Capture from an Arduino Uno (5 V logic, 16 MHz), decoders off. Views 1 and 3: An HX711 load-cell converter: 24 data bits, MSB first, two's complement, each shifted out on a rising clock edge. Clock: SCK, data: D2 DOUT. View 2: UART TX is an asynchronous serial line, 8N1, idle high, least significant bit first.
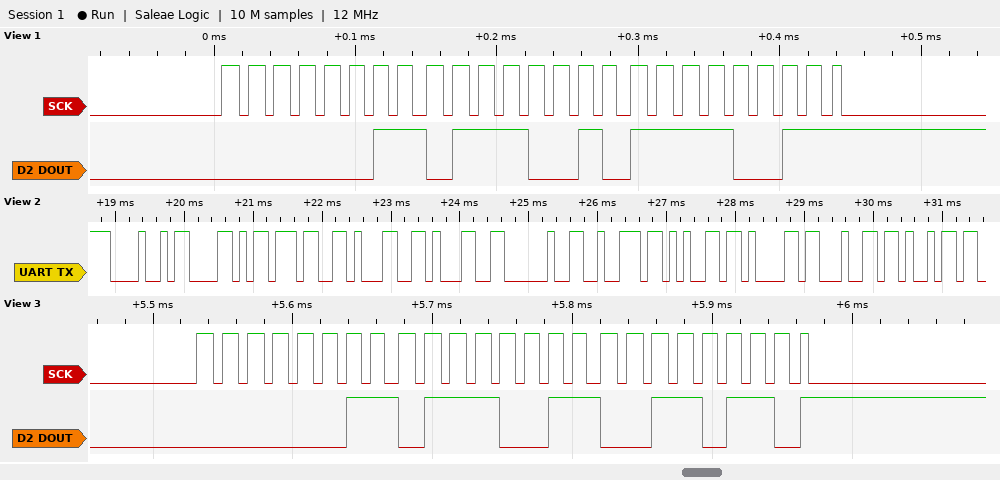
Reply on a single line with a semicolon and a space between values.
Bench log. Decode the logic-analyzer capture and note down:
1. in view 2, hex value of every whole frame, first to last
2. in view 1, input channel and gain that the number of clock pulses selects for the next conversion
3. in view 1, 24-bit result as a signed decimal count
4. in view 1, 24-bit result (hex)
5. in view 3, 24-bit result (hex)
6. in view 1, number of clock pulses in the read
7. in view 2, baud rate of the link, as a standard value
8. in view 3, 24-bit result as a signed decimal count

48 58 37 31 31 20 72 65 61 64 69; channel A, gain 128; 226035; 0x0372F3; 0x037336; 25; 9600 baud; 226102
